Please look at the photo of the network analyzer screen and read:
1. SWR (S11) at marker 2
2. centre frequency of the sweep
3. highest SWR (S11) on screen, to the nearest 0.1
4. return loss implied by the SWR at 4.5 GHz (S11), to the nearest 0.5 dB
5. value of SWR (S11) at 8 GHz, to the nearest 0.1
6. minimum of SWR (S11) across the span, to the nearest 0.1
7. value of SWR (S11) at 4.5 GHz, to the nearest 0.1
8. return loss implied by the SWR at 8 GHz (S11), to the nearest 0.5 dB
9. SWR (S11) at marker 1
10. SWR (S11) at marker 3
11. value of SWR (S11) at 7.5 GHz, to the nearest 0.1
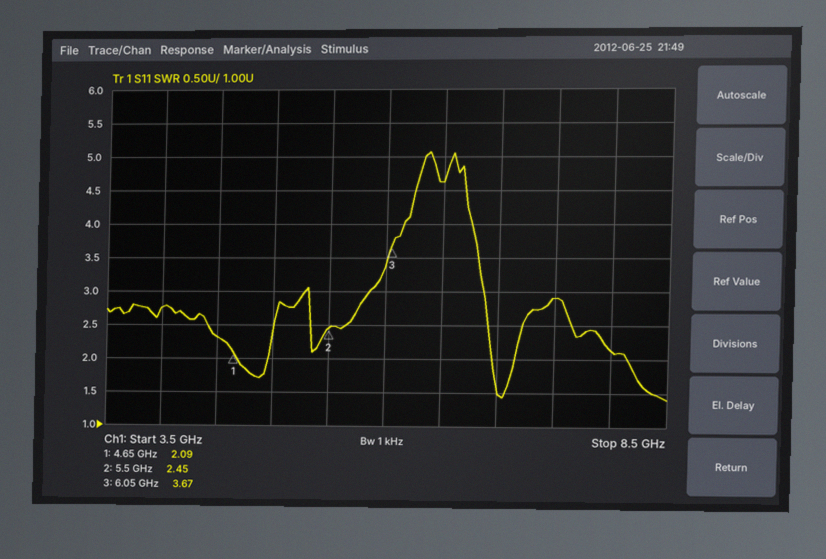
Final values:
2.45
6 GHz
5.1
8.0 dB
2.1
1.4
2.3
9.0 dB
2.09
3.67
2.9
